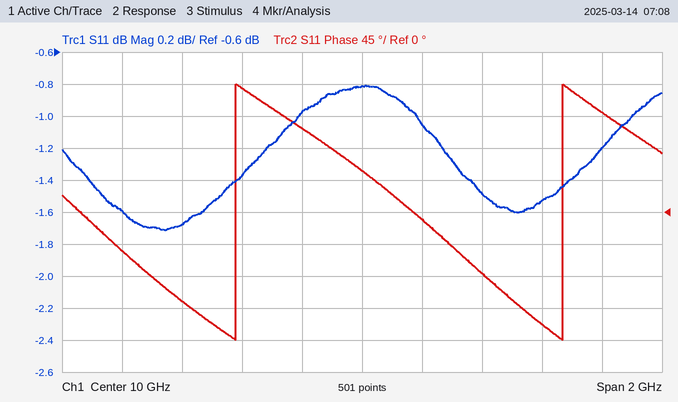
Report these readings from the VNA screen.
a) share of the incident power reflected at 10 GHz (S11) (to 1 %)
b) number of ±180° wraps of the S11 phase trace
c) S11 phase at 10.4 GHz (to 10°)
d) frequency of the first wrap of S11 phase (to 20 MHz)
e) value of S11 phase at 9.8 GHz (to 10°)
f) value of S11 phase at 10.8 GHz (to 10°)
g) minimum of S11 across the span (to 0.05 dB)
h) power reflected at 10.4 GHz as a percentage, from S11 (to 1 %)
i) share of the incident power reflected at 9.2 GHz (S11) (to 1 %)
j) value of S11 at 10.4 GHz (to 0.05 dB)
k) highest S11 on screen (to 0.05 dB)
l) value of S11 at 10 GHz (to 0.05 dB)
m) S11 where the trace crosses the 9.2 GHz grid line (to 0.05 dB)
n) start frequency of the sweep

83 %
2
-90°
9.58 GHz
120°
140°
-1.70 dB
71 %
69 %
-1.50 dB
-0.80 dB
-0.80 dB
-1.60 dB
9 GHz
